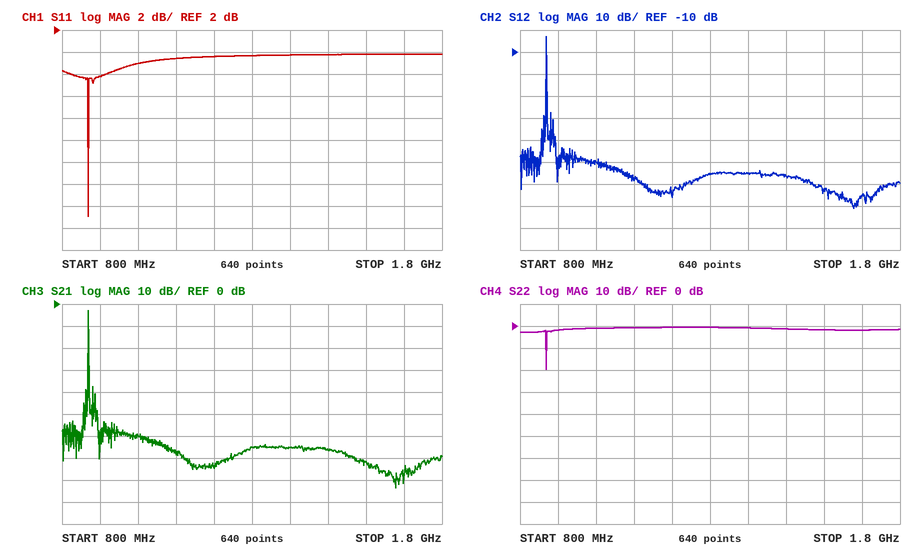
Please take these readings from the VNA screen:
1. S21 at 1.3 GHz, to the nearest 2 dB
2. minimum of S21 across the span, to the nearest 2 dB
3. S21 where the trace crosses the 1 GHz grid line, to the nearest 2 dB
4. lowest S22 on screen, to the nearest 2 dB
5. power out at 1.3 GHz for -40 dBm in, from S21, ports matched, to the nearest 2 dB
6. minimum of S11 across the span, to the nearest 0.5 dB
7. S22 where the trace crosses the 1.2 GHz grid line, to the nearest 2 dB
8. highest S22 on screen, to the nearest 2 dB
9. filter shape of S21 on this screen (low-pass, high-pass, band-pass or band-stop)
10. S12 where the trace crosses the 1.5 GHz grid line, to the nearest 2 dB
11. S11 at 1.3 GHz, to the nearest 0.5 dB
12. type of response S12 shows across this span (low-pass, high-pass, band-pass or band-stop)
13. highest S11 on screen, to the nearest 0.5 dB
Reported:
-66 dB
-84 dB
-60 dB
-20 dB
-106 dBm
-15.0 dB
0 dB
0 dB
band-pass
-66 dB
-0.5 dB
band-pass
0.0 dB
